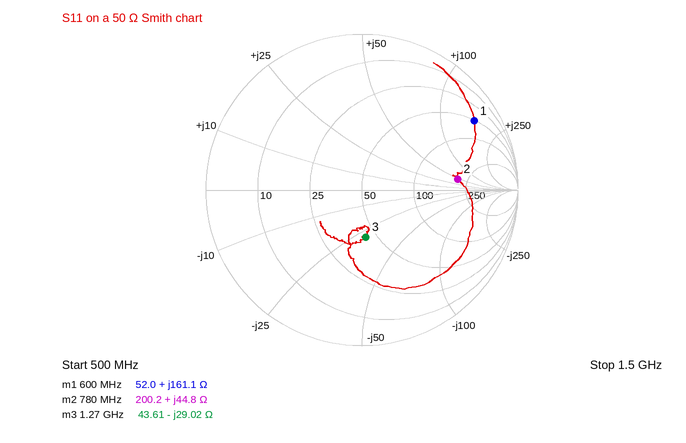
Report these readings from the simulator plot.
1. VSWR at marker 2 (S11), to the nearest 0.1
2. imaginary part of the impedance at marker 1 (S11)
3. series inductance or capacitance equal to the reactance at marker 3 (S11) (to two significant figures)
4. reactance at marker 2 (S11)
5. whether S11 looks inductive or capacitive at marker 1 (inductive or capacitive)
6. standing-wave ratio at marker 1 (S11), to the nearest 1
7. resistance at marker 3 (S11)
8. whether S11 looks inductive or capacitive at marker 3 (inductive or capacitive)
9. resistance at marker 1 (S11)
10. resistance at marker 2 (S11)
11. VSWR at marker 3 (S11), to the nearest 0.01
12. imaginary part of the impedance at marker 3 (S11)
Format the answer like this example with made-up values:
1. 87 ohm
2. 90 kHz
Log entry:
1. 4.2
2. +161.1 Ω
3. 4.3 pF
4. +44.8 Ω
5. inductive
6. 12
7. 43.61 Ω
8. capacitive
9. 52.0 Ω
10. 200.2 Ω
11. 1.87
12. -29.02 Ω
